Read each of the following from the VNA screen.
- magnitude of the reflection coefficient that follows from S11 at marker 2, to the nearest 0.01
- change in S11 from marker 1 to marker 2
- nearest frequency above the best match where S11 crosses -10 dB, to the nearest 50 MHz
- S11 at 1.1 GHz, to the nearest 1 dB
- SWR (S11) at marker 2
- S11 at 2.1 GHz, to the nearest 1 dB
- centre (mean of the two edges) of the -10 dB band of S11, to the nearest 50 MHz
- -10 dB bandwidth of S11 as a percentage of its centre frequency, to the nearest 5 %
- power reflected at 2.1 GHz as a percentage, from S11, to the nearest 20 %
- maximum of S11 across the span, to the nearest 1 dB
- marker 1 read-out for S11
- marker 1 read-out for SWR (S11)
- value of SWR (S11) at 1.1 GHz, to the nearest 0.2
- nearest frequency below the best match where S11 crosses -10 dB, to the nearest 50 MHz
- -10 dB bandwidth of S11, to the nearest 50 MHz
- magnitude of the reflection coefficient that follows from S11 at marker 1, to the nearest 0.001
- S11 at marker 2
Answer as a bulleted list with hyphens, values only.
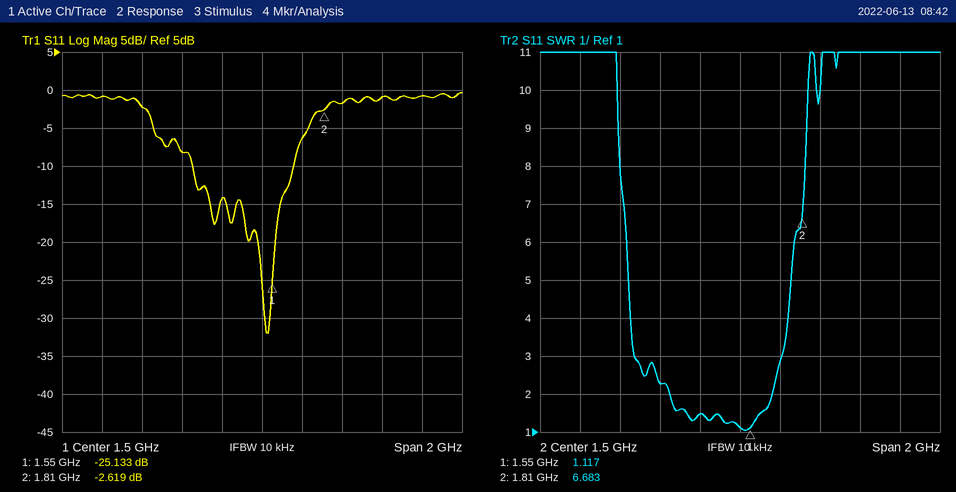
- 0.74
- 22.514 dB
- 1.65 GHz
- -8 dB
- 6.683
- -1 dB
- 1.40 GHz
- 35 %
- 80 %
- 0 dB
- -25.133 dB
- 1.117
- 2.2
- 1.15 GHz
- 500 MHz
- 0.055
- -2.619 dB
